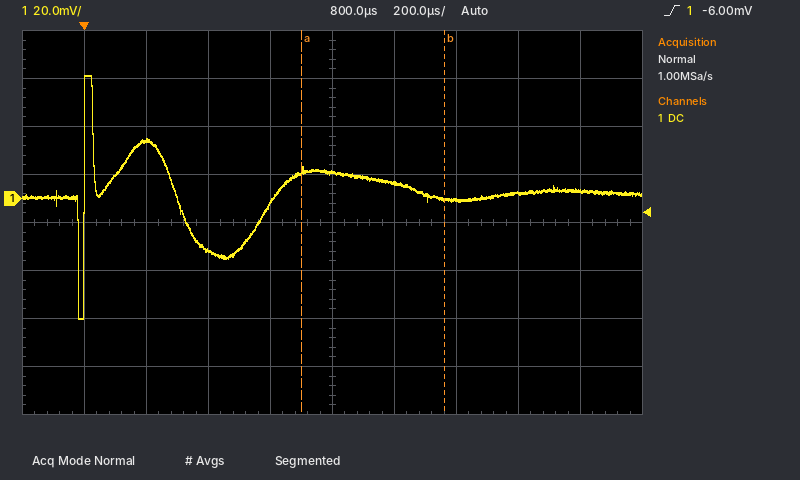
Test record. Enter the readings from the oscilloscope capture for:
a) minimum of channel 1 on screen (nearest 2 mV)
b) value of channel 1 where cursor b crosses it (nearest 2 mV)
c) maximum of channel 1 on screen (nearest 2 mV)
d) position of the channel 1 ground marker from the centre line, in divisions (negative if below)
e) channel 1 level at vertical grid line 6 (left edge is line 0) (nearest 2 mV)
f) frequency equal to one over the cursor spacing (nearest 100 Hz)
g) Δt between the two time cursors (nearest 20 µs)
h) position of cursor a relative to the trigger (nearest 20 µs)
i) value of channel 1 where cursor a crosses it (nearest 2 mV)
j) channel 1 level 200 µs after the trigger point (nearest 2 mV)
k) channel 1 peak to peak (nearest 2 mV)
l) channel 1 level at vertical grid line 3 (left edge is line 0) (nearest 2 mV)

-50 mV
0 mV
52 mV
+0.5 div
6 mV
2.2 kHz
460 µs
+700 µs
12 mV
24 mV
102 mV
-22 mV
